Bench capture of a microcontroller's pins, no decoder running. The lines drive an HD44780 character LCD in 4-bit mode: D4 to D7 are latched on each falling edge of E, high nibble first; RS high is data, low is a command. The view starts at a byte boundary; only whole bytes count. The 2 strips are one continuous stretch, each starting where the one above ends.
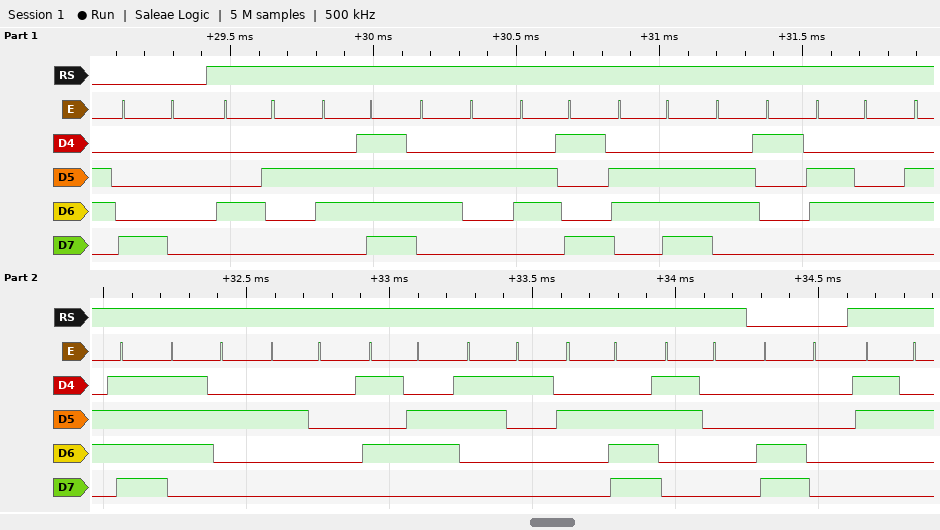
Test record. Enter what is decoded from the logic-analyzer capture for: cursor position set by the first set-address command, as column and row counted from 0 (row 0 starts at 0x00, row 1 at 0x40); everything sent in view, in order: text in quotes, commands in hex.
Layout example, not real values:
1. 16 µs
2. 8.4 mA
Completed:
1. column 0, row 0
2. 0x80 "Bobinador V1.0" 0xC0 "2"
